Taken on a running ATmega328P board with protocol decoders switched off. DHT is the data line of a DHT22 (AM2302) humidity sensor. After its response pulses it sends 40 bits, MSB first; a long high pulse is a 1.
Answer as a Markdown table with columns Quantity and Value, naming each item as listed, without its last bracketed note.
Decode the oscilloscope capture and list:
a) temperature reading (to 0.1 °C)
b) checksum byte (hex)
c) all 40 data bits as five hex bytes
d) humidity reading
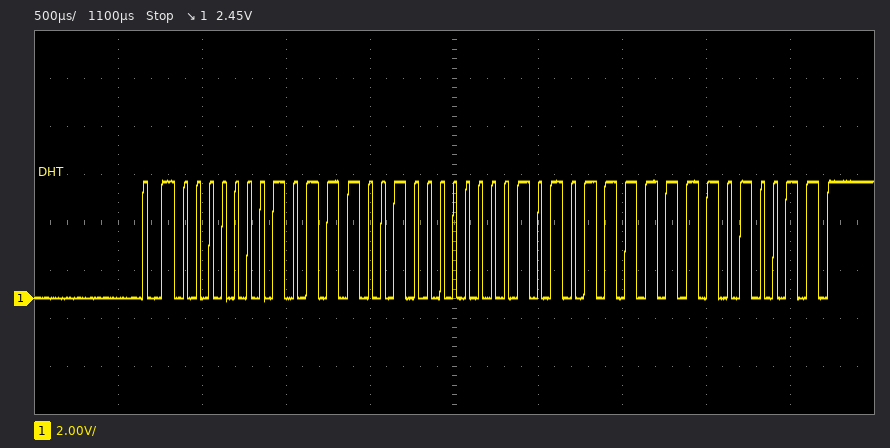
| Quantity | Value |
|---|---|
| temperature reading | 35.1 °C |
| checksum byte | 0xD3 |
| all 40 data bits as five hex bytes | 01 72 01 5F D3 |
| humidity reading | 37.0 % |
